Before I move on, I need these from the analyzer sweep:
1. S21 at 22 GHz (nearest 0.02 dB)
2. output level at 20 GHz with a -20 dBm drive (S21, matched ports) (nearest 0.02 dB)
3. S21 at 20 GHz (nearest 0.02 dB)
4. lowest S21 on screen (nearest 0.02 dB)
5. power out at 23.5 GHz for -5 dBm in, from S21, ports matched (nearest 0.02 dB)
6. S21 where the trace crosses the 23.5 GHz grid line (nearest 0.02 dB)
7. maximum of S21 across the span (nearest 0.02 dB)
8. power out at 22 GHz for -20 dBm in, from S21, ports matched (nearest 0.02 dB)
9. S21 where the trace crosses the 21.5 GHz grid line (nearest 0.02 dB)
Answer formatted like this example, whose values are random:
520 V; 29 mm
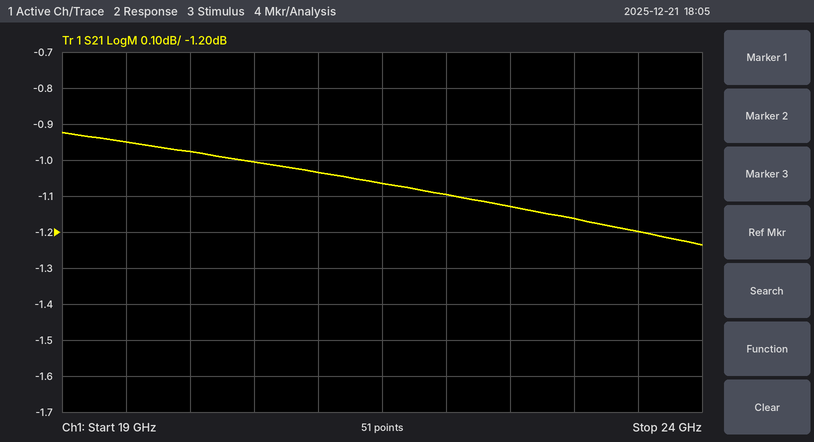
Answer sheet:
-1.10 dB; -20.98 dBm; -0.98 dB; -1.24 dB; -6.20 dBm; -1.20 dB; -0.92 dB; -21.10 dBm; -1.06 dB
